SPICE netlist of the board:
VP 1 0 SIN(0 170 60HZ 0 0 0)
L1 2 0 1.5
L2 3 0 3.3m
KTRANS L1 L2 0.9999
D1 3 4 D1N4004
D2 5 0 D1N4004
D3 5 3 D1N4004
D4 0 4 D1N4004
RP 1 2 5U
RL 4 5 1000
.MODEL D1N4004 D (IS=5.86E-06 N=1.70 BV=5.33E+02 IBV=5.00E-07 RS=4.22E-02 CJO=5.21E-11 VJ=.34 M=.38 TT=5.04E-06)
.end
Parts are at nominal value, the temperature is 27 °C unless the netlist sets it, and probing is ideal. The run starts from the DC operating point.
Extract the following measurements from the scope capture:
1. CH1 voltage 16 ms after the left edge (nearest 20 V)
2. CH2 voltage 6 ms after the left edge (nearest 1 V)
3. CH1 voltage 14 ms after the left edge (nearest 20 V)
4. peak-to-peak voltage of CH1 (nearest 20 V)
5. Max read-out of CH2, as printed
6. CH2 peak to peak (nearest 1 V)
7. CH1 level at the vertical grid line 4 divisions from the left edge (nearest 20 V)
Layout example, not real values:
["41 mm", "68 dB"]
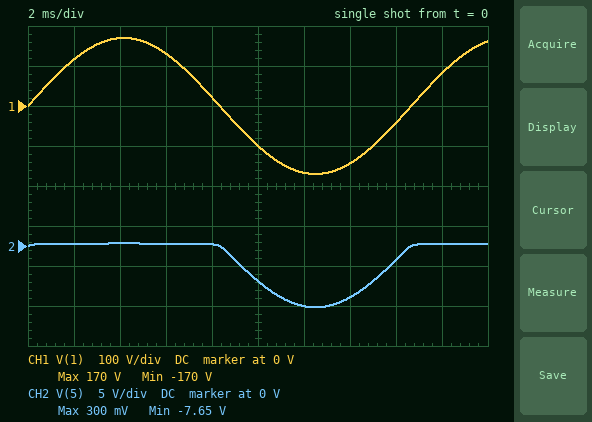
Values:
["-40 V", "0 V", "-140 V", "340 V", "300 mV", "8 V", "20 V"]
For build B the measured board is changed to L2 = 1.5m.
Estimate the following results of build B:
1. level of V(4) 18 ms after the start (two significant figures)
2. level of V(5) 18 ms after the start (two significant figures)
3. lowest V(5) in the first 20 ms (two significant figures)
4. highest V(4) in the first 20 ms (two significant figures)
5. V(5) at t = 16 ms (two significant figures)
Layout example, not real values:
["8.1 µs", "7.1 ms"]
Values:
["2.3 V", "260 mV", "-5.1 V", "5.1 V", "-1.1 V"]
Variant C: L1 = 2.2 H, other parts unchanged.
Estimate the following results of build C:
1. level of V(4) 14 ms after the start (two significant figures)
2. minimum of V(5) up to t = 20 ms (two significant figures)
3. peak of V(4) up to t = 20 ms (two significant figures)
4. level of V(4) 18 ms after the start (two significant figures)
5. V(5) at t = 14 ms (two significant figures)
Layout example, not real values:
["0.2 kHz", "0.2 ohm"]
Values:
["-300 mV", "-6.3 V", "6.3 V", "2.9 V", "-5.3 V"]
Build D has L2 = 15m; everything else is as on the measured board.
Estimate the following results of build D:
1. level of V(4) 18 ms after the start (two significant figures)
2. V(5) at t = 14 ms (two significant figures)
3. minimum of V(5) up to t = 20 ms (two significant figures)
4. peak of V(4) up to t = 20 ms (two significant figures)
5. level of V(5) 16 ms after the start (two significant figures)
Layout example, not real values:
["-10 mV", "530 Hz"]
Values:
["7.9 V", "-14 V", "-17 V", "17 V", "-3.9 V"]
